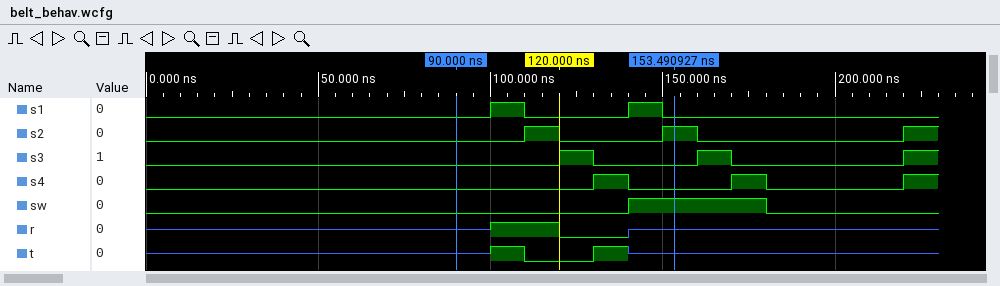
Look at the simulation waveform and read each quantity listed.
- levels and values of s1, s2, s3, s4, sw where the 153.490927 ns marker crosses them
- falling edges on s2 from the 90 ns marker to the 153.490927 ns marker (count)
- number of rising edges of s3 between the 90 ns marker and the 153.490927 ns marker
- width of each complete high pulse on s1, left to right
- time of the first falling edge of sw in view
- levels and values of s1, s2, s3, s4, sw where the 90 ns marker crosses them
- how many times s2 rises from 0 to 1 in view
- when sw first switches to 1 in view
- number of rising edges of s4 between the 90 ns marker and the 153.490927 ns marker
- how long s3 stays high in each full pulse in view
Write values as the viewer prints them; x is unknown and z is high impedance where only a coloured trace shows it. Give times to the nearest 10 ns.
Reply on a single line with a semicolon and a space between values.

s1=0, s2=1, s3=0, s4=0, sw=1; 1; 1; 10 ns, 10 ns; 180 ns; s1=0, s2=0, s3=0, s4=0, sw=0; 3; 140 ns; 1; 10 ns, 10 ns
